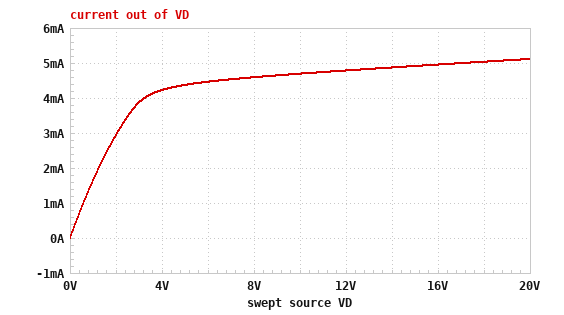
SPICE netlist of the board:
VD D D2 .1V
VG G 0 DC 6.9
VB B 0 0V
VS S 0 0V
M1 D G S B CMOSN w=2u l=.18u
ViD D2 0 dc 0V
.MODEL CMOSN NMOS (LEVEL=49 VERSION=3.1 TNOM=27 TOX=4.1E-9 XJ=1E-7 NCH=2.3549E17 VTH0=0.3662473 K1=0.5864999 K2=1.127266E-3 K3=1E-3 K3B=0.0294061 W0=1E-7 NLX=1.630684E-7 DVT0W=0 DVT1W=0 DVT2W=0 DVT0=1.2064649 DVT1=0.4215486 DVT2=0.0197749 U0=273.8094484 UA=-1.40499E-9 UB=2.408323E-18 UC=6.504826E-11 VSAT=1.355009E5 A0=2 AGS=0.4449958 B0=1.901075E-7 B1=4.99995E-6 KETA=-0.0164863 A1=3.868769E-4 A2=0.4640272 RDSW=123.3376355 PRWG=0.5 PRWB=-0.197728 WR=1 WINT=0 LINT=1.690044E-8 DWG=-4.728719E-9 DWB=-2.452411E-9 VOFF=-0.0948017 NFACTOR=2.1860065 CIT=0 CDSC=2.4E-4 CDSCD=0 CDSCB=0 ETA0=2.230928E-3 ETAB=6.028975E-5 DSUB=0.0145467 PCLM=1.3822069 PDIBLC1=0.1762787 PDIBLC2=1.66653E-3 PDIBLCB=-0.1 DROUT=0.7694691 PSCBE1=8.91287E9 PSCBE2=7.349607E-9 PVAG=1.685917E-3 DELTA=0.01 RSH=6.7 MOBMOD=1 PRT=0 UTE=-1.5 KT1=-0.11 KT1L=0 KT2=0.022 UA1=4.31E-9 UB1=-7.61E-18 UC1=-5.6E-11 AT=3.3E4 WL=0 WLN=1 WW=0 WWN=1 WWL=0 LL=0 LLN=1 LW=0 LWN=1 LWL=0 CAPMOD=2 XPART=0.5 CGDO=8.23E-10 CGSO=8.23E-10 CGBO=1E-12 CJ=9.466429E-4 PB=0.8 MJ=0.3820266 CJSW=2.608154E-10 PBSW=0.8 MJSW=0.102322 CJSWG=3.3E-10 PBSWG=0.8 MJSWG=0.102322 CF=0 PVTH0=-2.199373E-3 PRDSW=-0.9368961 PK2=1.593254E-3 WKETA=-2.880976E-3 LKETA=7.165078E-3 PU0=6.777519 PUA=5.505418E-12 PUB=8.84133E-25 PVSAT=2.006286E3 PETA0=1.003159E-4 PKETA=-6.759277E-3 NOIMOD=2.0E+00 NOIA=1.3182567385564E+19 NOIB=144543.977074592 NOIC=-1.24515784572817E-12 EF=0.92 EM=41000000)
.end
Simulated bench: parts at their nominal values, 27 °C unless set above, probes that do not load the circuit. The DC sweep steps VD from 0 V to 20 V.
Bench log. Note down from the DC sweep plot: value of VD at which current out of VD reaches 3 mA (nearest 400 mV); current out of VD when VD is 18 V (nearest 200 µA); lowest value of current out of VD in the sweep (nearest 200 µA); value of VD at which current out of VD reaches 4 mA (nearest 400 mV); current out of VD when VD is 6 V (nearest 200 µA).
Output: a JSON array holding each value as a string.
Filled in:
["2.0 V", "5.0 mA", "0 A", "3.2 V", "4.4 mA"]
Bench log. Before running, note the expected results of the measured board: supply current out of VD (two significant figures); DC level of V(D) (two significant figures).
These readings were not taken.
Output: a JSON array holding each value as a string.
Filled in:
["180 µA", "100 mV"]
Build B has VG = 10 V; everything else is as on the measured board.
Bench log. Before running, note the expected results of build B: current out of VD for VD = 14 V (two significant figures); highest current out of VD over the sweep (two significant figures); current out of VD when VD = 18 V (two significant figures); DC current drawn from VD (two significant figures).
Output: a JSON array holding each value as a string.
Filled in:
["6.1 mA", "6.4 mA", "6.3 mA", "130 µA"]
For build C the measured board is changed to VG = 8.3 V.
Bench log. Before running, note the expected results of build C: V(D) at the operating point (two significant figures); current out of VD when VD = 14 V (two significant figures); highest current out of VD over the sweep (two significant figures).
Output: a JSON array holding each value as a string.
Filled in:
["100 mV", "5.5 mA", "5.7 mA"]
